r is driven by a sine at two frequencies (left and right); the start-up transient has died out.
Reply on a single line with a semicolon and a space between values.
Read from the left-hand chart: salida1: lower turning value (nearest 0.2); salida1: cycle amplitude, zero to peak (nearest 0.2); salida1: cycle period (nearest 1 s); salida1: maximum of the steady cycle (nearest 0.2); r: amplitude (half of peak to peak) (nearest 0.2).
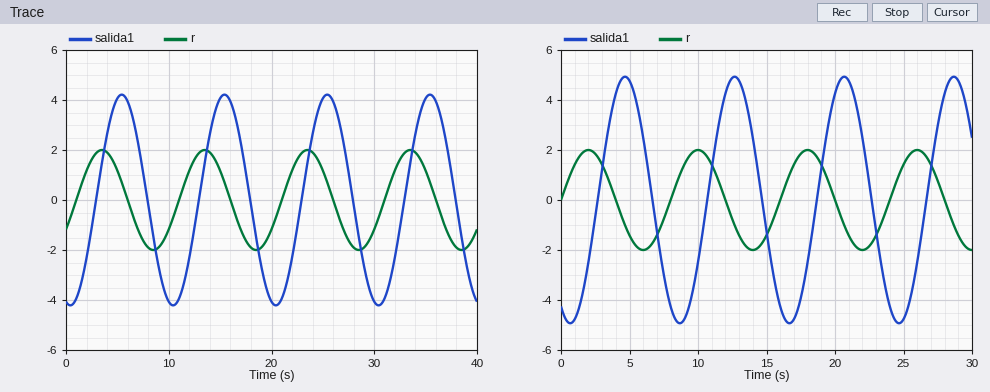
-4.2; 4.2; 10 s; 4.2; 2.0
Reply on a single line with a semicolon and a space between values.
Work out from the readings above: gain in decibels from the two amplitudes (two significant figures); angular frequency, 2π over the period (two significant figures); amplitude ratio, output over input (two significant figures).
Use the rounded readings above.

6.4 dB; 0.63 rad/s; 2.1
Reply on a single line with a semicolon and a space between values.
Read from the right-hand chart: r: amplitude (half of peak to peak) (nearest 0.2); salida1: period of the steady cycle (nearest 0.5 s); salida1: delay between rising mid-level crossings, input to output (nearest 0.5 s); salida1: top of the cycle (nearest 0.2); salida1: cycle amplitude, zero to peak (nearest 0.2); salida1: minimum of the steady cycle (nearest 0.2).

2.0; 8.0 s; 2.5 s; 5.0; 5.0; -5.0
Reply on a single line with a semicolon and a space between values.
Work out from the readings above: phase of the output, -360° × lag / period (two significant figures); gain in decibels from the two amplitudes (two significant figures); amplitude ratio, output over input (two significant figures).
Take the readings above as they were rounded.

-110°; 8.0 dB; 2.5
